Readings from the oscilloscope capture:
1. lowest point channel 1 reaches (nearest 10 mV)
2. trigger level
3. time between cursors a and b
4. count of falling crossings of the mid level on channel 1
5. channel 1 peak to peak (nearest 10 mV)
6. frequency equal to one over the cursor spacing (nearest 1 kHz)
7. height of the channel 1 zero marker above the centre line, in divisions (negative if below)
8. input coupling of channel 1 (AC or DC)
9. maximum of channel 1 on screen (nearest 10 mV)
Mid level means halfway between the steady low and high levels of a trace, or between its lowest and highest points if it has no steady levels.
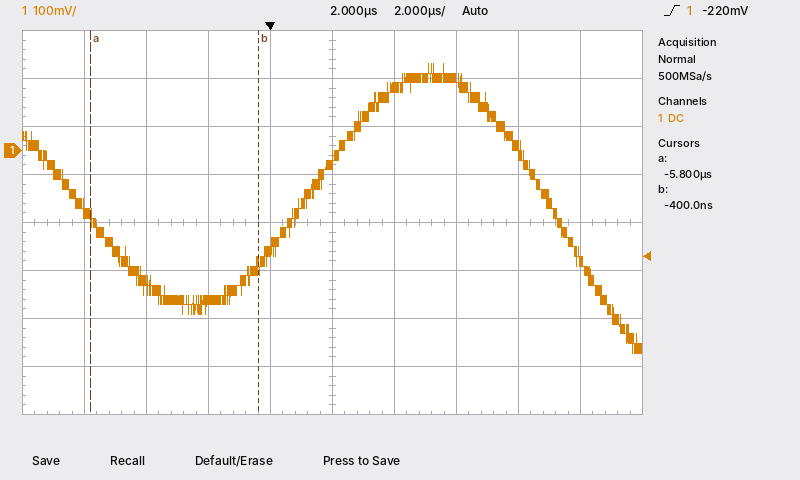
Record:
-420 mV
-220 mV
5.4 µs
2
600 mV
185 kHz
+1.5 div
DC
180 mV
